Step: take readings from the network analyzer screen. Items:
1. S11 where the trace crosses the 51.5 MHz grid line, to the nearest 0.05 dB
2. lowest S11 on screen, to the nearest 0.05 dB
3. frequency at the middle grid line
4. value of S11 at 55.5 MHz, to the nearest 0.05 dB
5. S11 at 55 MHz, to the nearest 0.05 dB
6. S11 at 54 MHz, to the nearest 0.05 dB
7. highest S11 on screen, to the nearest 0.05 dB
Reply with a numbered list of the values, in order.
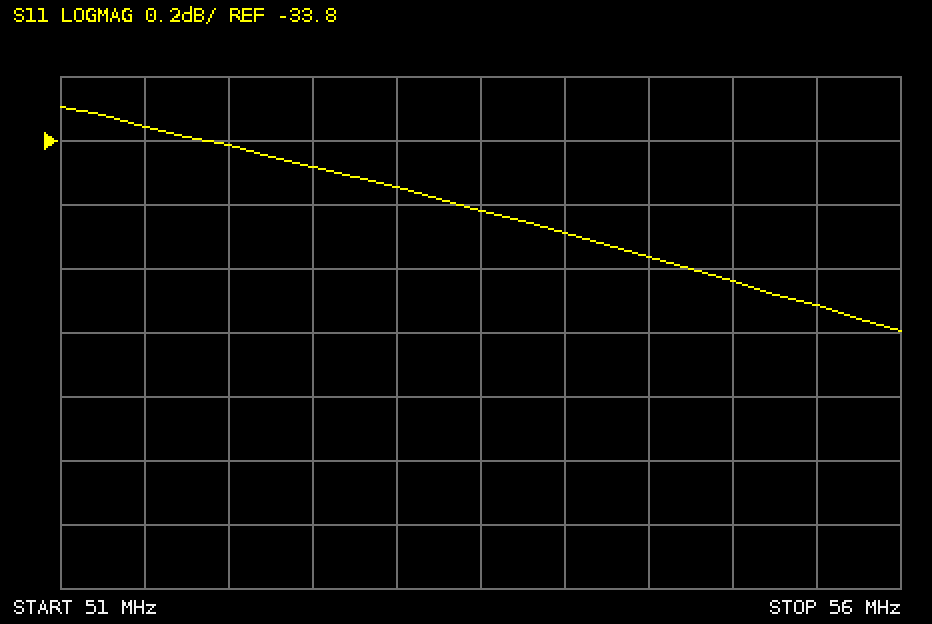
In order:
1. -33.75 dB
2. -34.40 dB
3. 53.5 MHz
4. -34.30 dB
5. -34.25 dB
6. -34.10 dB
7. -33.70 dB
